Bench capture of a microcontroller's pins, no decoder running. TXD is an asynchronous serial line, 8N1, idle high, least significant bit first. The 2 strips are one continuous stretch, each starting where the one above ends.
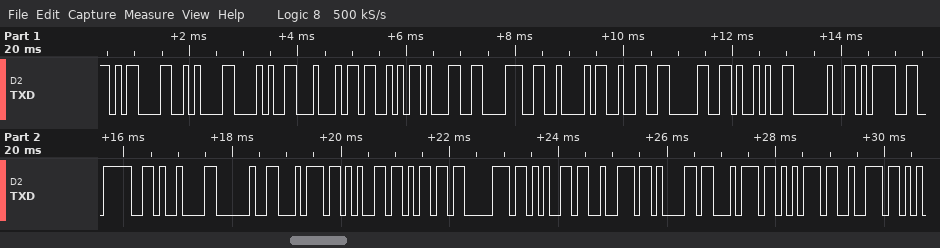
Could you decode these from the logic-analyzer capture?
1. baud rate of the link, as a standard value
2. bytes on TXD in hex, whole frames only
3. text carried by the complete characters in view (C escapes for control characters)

9600 baud
0D 0A 28 44 53 31 38 42 32 30 29 20 3D 3E 09 20 74 65 6D 70 65 72 61 74 75 72
"\r\n(DS18B20) =>\t temperatur"
